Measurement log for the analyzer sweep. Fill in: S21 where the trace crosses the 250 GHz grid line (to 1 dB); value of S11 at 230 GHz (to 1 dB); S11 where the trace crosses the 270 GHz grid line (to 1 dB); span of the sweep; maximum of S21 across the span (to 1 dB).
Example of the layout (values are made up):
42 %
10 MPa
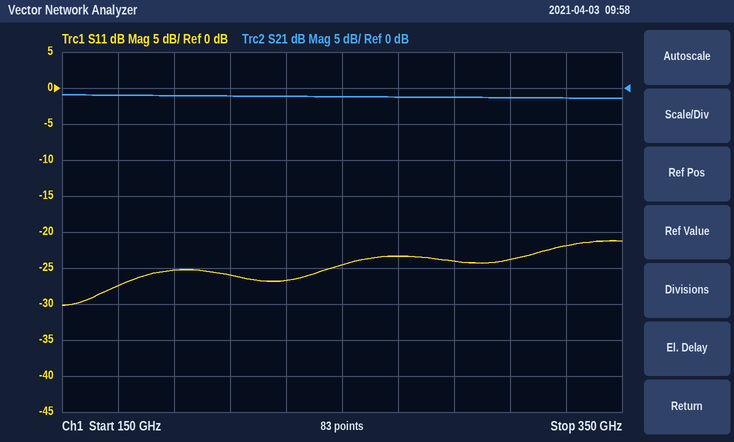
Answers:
-1 dB
-27 dB
-23 dB
200 GHz
-1 dB
